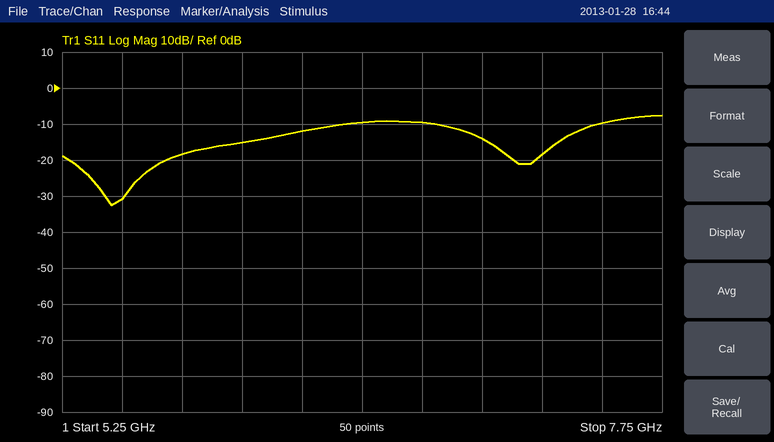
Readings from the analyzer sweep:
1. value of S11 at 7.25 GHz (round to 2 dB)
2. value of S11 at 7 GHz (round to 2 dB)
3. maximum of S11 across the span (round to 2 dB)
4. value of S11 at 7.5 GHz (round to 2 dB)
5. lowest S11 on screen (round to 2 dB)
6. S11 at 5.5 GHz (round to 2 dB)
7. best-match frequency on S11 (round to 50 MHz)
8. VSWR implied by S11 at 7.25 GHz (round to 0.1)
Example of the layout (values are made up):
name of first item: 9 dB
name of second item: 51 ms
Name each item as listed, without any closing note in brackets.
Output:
value of S11 at 7.25 GHz: -18 dB
value of S11 at 7 GHz: -14 dB
maximum of S11 across the span: -8 dB
value of S11 at 7.5 GHz: -10 dB
lowest S11 on screen: -32 dB
S11 at 5.5 GHz: -30 dB
best-match frequency on S11: 5.45 GHz
VSWR implied by S11 at 7.25 GHz: 1.3
